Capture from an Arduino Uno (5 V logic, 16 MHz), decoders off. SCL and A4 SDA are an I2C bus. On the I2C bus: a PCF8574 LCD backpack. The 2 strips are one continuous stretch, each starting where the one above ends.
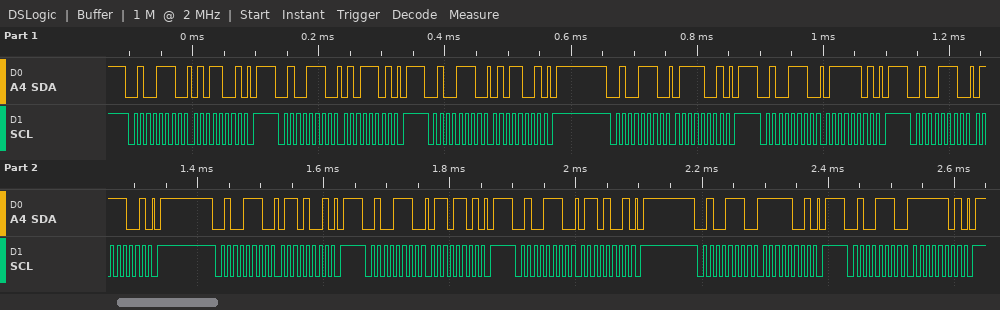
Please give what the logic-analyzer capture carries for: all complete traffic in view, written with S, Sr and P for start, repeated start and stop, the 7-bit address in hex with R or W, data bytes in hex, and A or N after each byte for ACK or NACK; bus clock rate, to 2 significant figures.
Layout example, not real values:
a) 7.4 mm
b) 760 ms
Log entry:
a) S 27W A 59 A P S 27W A 5D A P S 27W A 59 A P S 27W A 79 A P S 27W A 7D A P S 27W A 79 A P S 27W A 69 A P S 27W A 6D A P S 27W A 69 A P S 27W A F9 A P S 27W A FD A P
b) 100 kHz
